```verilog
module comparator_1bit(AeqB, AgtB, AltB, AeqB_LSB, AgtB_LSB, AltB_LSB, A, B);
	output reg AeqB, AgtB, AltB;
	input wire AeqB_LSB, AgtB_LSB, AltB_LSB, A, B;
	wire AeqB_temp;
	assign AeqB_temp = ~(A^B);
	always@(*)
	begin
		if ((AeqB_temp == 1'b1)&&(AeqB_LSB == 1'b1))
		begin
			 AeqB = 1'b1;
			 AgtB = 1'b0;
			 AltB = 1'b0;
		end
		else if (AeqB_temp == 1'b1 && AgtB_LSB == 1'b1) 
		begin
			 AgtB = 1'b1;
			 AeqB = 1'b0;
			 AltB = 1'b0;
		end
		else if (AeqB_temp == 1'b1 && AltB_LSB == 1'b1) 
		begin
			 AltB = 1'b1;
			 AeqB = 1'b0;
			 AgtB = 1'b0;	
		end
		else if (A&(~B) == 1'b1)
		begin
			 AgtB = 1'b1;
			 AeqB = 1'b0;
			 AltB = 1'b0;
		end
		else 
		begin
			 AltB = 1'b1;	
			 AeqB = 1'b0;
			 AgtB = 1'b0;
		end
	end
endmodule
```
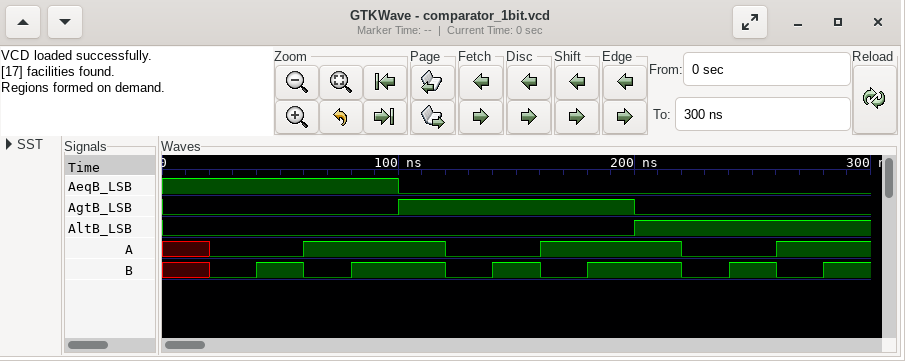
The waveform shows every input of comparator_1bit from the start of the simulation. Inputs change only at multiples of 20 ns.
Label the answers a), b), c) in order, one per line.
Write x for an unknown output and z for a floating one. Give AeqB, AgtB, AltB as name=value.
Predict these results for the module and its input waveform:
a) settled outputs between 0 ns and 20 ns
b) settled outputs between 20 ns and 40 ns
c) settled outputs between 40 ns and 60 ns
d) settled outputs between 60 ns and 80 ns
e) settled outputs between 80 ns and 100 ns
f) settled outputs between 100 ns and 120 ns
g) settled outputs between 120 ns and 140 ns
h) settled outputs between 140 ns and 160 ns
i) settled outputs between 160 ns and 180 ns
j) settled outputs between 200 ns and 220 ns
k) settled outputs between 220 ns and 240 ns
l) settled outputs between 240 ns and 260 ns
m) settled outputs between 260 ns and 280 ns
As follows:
a) AeqB=0, AgtB=0, AltB=1
b) AeqB=1, AgtB=0, AltB=0
c) AeqB=0, AgtB=0, AltB=1
d) AeqB=0, AgtB=1, AltB=0
e) AeqB=1, AgtB=0, AltB=0
f) AeqB=0, AgtB=1, AltB=0
g) AeqB=0, AgtB=1, AltB=0
h) AeqB=0, AgtB=0, AltB=1
i) AeqB=0, AgtB=1, AltB=0
j) AeqB=0, AgtB=0, AltB=1
k) AeqB=0, AgtB=0, AltB=1
l) AeqB=0, AgtB=0, AltB=1
m) AeqB=0, AgtB=1, AltB=0
